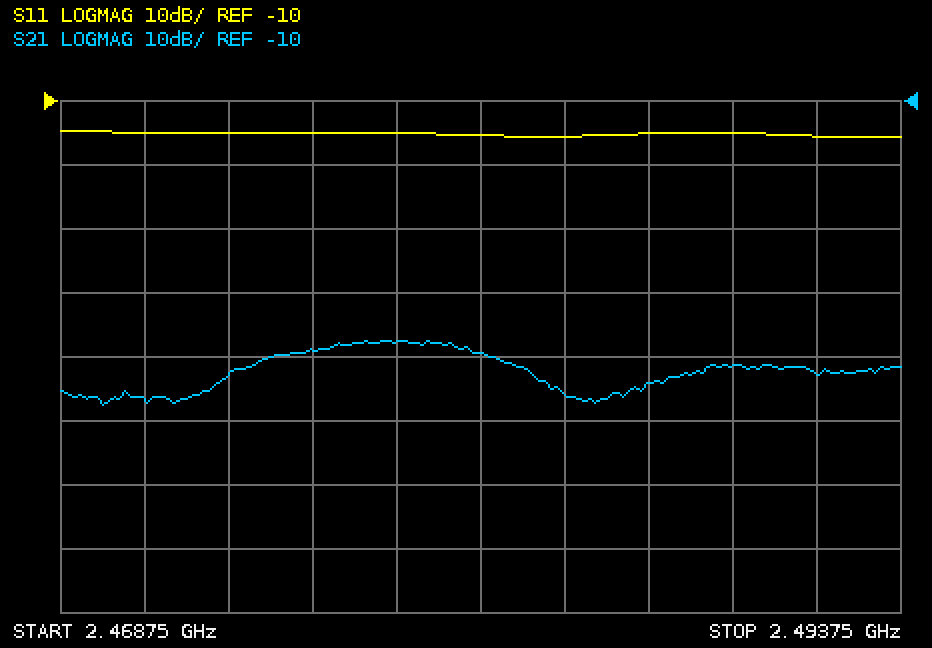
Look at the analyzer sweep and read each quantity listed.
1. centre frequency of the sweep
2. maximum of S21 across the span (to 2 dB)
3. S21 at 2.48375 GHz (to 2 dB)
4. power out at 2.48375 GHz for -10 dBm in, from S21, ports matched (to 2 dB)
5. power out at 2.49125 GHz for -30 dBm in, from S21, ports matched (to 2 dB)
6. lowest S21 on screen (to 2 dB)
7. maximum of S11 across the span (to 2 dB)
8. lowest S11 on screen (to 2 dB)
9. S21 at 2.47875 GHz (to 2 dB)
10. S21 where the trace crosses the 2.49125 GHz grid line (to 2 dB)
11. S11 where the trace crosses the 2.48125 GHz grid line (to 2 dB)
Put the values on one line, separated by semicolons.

2.48125 GHz; -48 dB; -56 dB; -66 dBm; -82 dBm; -58 dB; -14 dB; -16 dB; -48 dB; -52 dB; -16 dB
